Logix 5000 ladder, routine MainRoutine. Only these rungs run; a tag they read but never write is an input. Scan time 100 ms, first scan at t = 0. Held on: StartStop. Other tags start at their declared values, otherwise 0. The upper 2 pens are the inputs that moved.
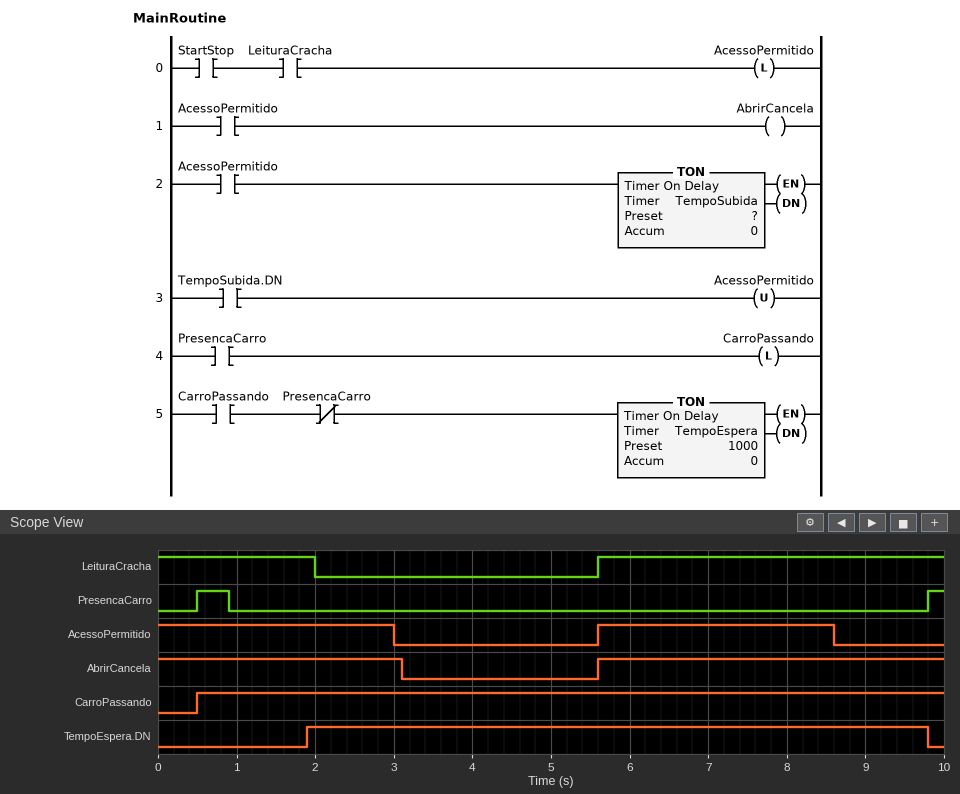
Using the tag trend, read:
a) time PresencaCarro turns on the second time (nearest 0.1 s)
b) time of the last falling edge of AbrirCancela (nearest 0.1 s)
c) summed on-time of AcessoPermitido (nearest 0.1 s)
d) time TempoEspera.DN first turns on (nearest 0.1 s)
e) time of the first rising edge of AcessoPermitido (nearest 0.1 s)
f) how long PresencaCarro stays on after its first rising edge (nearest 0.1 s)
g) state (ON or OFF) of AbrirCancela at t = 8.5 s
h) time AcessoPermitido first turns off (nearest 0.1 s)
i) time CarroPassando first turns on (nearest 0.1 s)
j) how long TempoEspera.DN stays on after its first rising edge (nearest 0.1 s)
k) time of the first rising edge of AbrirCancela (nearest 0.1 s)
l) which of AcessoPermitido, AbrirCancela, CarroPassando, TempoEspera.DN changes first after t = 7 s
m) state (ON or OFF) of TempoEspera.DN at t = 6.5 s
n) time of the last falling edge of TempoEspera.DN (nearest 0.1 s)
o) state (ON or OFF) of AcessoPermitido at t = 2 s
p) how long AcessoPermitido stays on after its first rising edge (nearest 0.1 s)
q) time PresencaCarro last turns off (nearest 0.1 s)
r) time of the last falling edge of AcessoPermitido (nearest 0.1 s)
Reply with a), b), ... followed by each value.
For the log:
a) 9.8 s
b) 3.1 s
c) 6.0 s
d) 1.9 s
e) 5.6 s
f) 0.4 s
g) ON
h) 3.0 s
i) 0.5 s
j) 7.9 s
k) 5.6 s
l) AcessoPermitido
m) ON
n) 9.8 s
o) ON
p) 3.0 s
q) 0.9 s
r) 8.6 s
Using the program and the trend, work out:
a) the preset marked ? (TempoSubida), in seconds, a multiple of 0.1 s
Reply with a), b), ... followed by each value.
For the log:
a) 3.0 s
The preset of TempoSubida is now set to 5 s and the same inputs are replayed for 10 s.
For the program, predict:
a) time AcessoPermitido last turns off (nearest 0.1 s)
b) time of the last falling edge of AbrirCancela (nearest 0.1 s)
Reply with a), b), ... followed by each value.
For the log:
a) 5.0 s
b) 5.1 s
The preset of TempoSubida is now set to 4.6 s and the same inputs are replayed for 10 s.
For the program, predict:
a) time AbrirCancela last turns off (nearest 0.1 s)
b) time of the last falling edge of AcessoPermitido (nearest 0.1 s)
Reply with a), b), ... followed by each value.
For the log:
a) 4.7 s
b) 4.6 s
